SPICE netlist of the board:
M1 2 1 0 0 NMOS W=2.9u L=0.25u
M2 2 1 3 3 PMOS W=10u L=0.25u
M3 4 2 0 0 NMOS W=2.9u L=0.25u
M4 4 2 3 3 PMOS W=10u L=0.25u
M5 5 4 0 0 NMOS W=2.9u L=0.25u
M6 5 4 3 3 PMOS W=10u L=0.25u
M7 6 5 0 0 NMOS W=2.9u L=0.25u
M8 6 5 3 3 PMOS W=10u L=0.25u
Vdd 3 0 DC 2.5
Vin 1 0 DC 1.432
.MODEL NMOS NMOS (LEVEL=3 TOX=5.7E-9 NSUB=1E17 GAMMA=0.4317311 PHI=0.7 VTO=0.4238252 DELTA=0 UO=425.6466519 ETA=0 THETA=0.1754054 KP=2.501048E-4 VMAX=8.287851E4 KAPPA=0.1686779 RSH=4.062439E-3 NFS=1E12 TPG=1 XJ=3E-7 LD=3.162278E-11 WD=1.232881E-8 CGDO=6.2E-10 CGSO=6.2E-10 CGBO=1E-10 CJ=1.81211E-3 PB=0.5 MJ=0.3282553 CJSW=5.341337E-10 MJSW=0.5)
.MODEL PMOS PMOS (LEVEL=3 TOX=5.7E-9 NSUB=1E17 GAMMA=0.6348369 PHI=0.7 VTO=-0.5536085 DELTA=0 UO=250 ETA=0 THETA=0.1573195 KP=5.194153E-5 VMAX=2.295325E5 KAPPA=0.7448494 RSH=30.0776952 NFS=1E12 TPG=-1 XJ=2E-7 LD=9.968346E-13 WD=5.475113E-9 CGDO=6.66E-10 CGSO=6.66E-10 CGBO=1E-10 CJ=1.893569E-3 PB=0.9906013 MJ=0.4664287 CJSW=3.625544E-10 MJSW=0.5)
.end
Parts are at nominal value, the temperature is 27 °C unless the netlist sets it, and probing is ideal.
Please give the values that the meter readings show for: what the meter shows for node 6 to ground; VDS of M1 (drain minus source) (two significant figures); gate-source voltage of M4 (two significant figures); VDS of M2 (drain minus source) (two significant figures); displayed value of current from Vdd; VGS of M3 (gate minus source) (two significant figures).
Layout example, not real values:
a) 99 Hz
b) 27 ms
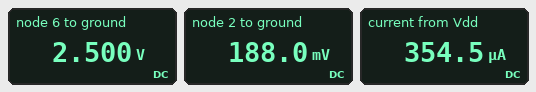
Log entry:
a) 2.500 V
b) 190 mV
c) -2.3 V
d) -2.3 V
e) 354.5 µA
f) 190 mV
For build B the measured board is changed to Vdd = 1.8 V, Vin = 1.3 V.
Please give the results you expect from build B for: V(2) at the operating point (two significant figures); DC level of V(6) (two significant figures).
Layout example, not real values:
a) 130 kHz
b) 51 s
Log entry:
a) 5.6 mV
b) 1.8 V
